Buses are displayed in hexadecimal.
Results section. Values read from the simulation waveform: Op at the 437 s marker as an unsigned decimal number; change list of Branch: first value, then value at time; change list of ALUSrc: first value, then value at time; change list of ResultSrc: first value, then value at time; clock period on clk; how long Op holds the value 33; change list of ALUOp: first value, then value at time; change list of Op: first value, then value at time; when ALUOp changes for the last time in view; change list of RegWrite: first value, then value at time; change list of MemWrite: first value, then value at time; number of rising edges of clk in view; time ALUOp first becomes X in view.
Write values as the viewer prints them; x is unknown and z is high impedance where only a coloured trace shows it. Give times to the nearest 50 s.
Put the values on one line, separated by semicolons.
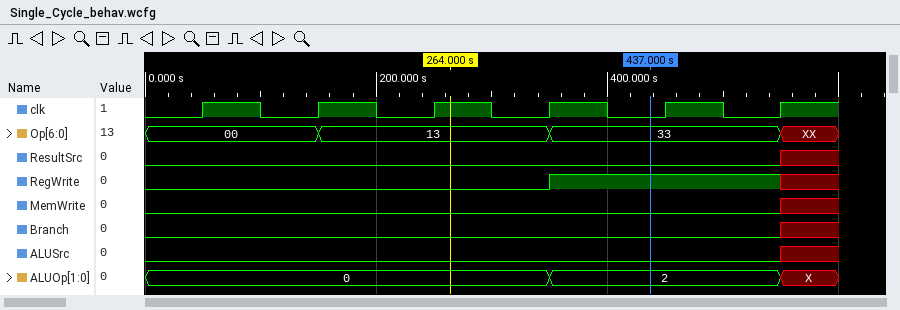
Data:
51; 0, x at 550 s; 0, x at 550 s; 0, x at 550 s; 100 s; 200 s; 0, 2 at 350 s, X at 550 s; 00, 13 at 150 s, 33 at 350 s, XX at 550 s; 550 s; 0, 1 at 350 s, x at 550 s; 0, x at 550 s; 6; 550 s
